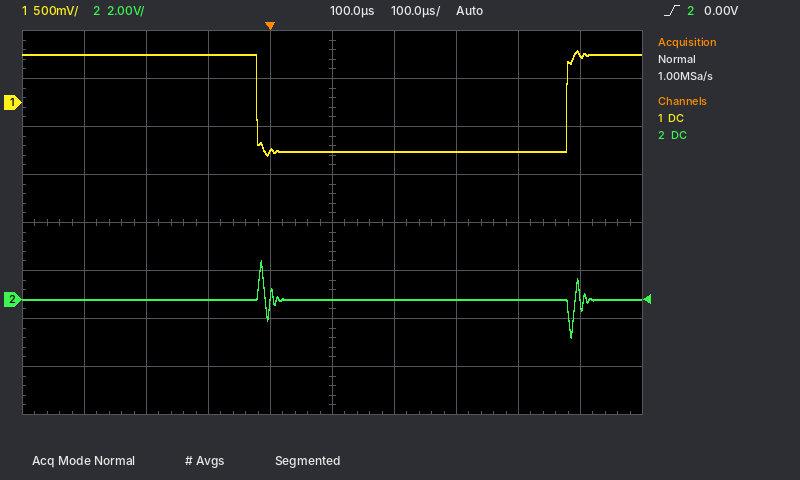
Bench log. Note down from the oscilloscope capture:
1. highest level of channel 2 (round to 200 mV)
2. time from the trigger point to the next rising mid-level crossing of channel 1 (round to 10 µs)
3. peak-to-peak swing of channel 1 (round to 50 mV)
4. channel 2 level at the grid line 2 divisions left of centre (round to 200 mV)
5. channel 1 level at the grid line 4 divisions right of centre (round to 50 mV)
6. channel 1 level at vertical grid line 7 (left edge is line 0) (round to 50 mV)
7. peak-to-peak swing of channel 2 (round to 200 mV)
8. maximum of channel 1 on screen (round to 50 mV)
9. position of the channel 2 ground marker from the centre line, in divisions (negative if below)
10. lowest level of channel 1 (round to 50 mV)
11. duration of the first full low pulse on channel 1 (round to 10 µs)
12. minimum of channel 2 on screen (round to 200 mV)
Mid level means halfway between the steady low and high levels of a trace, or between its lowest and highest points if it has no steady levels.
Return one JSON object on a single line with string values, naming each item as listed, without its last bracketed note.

{"highest level of channel 2": "1.6 V", "time from the trigger point to the next rising mid-level crossing of channel 1": "480 µs", "peak-to-peak swing of channel 1": "1.10 V", "channel 2 level at the grid line 2 divisions left of centre": "0.0 V", "channel 1 level at the grid line 4 divisions right of centre": "500 mV", "channel 1 level at vertical grid line 7 (left edge is line 0)": "-500 mV", "peak-to-peak swing of channel 2": "3.2 V", "maximum of channel 1 on screen": "550 mV", "position of the channel 2 ground marker from the centre line, in divisions": "-1.6 div", "lowest level of channel 1": "-550 mV", "duration of the first full low pulse on channel 1": "500 µs", "minimum of channel 2 on screen": "-1.6 V"}
